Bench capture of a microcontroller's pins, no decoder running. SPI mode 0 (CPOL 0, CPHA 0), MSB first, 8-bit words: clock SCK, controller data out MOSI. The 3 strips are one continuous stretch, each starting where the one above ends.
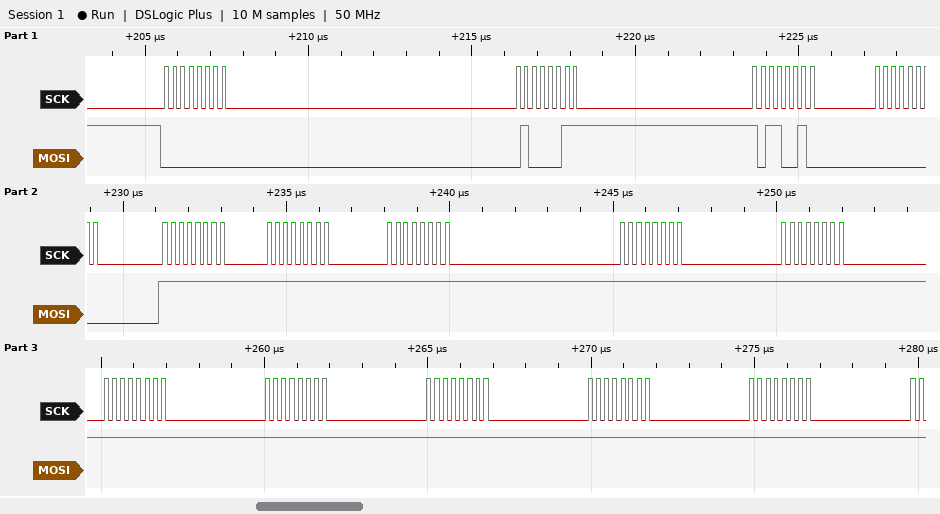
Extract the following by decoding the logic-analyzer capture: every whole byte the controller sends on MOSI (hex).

0x00 0x43 0xB2 0x00 0xFF 0xFF 0xFF 0xFF 0xFF 0xFF 0xFF 0xFF 0xFF 0xFF
